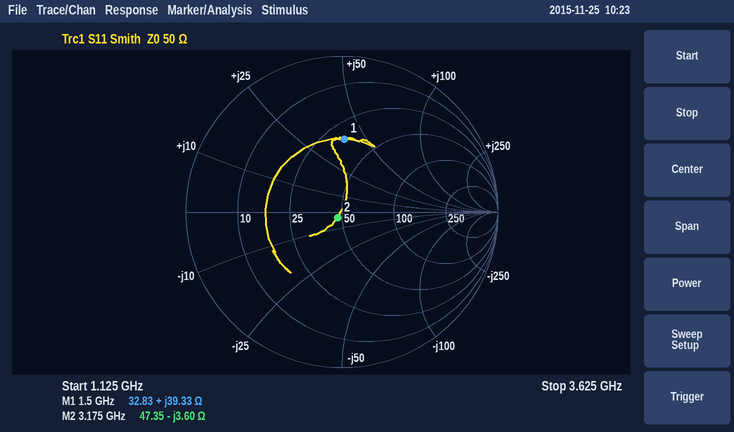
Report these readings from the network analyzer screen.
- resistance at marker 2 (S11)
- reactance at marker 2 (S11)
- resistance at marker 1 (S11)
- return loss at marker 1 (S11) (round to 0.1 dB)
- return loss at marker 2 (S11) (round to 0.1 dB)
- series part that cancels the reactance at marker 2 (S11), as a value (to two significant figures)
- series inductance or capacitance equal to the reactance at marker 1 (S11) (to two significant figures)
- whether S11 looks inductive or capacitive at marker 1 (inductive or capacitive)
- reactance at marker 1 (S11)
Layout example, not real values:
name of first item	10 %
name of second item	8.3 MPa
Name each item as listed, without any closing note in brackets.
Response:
resistance at marker 2	47.35 Ω
reactance at marker 2	-3.60 Ω
resistance at marker 1	32.83 Ω
return loss at marker 1 (S11)	6.6 dB
return loss at marker 2 (S11)	26.8 dB
series part that cancels the reactance at marker 2 (S11), as a value	180 pH
series inductance or capacitance equal to the reactance at marker 1 (S11)	4.2 nH
whether S11 looks inductive or capacitive at marker 1	inductive
reactance at marker 1	+39.33 Ω
